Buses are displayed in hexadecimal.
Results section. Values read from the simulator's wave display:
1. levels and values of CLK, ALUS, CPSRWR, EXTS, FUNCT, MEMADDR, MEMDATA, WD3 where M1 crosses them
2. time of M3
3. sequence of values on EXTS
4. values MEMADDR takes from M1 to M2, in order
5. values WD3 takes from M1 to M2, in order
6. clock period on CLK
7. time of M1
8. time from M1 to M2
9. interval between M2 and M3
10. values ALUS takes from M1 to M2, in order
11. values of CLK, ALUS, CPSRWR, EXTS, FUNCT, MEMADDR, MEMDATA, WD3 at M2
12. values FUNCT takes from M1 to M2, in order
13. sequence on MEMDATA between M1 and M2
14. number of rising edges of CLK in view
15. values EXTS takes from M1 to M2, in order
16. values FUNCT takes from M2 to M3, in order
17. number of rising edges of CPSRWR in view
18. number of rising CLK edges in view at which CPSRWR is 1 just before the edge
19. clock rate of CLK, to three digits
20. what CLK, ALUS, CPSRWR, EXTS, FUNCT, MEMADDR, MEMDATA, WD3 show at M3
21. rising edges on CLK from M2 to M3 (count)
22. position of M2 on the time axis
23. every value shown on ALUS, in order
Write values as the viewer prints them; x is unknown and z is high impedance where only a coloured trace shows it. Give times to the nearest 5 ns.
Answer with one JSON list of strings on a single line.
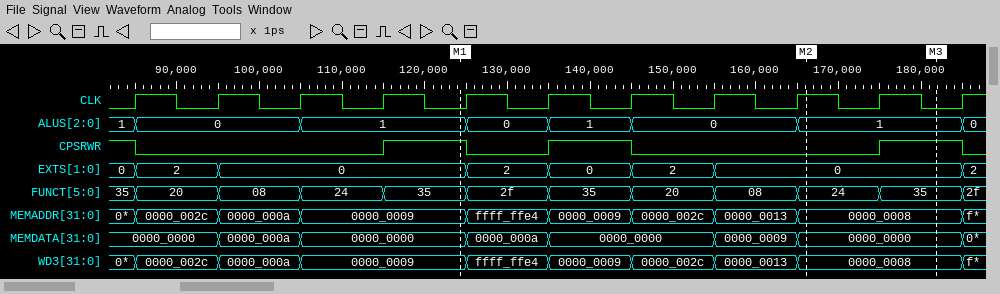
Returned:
["CLK=0, ALUS=1, CPSRWR=1, EXTS=0, FUNCT=35, MEMADDR=0000_0009, MEMDATA=0000_0000, WD3=0000_0009", "180 ns", "0, 2, 0, 2, 0, 2, 0, 2", "0000_0009, ffff_ffe4, 0000_0009, 0000_002c, 0000_0013, 0000_0008", "0000_0009, ffff_ffe4, 0000_0009, 0000_002c, 0000_0013, 0000_0008", "10 ns", "125 ns", "40 ns", "15 ns", "1, 0, 1, 0, 1", "CLK=1, ALUS=1, CPSRWR=0, EXTS=0, FUNCT=24, MEMADDR=0000_0008, MEMDATA=0000_0000, WD3=0000_0008", "35, 2f, 35, 20, 08, 24", "0000_0000, 0000_000a, 0000_0000, 0000_0009, 0000_0000", "11", "0, 2, 0, 2, 0", "24, 35", "3", "4", "100 MHz", "CLK=0, ALUS=1, CPSRWR=1, EXTS=0, FUNCT=35, MEMADDR=0000_0008, MEMDATA=0000_0000, WD3=0000_0008", "1", "165 ns", "1, 0, 1, 0, 1, 0, 1, 0"]
